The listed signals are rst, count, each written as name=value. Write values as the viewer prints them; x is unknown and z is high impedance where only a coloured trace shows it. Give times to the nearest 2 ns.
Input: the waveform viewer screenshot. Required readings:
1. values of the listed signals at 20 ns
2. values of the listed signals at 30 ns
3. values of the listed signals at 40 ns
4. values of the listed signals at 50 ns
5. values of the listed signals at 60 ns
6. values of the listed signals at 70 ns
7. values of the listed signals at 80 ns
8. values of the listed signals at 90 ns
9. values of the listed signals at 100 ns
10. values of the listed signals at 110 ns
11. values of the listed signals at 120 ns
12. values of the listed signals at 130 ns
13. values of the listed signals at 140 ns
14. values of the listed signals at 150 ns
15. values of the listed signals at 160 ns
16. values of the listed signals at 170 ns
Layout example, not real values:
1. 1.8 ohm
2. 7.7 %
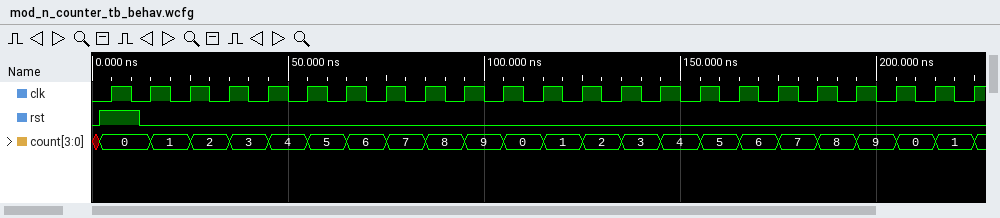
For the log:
1. rst=0, count=1
2. rst=0, count=2
3. rst=0, count=3
4. rst=0, count=4
5. rst=0, count=5
6. rst=0, count=6
7. rst=0, count=7
8. rst=0, count=8
9. rst=0, count=9
10. rst=0, count=0
11. rst=0, count=1
12. rst=0, count=2
13. rst=0, count=3
14. rst=0, count=4
15. rst=0, count=5
16. rst=0, count=6
